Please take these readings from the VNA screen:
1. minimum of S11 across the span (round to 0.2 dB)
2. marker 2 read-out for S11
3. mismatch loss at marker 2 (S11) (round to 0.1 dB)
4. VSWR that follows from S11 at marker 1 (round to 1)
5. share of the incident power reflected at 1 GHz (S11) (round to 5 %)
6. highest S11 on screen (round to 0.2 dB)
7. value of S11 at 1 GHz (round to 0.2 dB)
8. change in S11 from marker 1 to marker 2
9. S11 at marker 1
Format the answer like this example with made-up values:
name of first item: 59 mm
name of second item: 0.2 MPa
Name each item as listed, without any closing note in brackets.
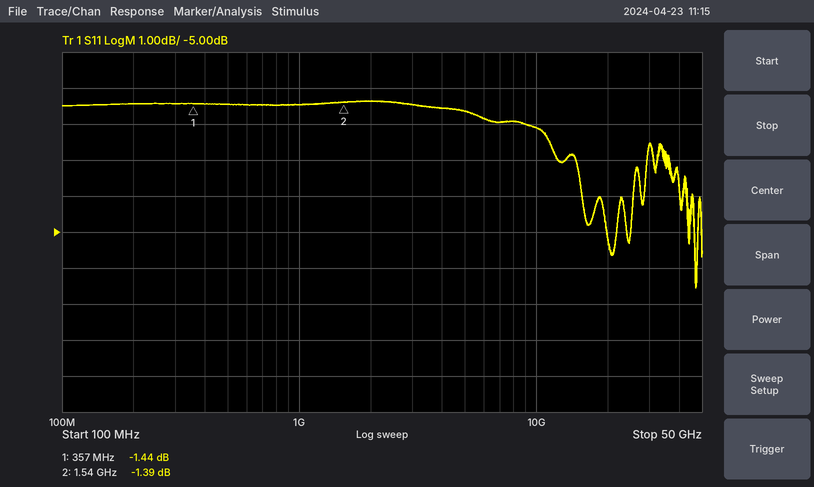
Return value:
minimum of S11 across the span: -6.6 dB
marker 2 read-out for S11: -1.39 dB
mismatch loss at marker 2 (S11): 5.6 dB
VSWR that follows from S11 at marker 1: 12
share of the incident power reflected at 1 GHz (S11): 70 %
highest S11 on screen: -1.4 dB
value of S11 at 1 GHz: -1.4 dB
change in S11 from marker 1 to marker 2: 0.05 dB
S11 at marker 1: -1.44 dB
